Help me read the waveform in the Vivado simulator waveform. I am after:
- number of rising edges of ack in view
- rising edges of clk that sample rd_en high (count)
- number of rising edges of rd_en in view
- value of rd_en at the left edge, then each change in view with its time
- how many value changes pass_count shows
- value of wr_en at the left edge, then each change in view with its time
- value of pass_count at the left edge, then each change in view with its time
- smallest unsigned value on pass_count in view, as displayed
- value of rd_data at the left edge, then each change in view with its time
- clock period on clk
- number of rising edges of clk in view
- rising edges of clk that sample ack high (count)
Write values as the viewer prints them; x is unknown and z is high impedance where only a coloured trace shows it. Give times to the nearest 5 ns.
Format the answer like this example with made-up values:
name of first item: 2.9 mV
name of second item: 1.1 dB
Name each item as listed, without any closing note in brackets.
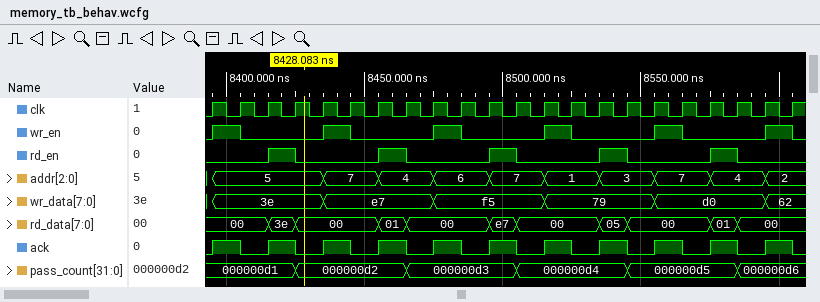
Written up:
number of rising edges of ack in view: 11
rising edges of clk that sample rd_en high: 5
number of rising edges of rd_en in view: 5
value of rd_en at the left edge, then each change in view with its time: 0, 1 at 8415 ns, 0 at 8425 ns, 1 at 8455 ns, 0 at 8465 ns, 1 at 8495 ns, 0 at 8505 ns, 1 at 8535 ns, 0 at 8545 ns, 1 at 8575 ns, 0 at 8585 ns
how many value changes pass_count shows: 5
value of wr_en at the left edge, then each change in view with its time: 0, 1 at 8395 ns, 0 at 8405 ns, 1 at 8435 ns, 0 at 8445 ns, 1 at 8475 ns, 0 at 8485 ns, 1 at 8515 ns, 0 at 8525 ns, 1 at 8555 ns, 0 at 8565 ns, 1 at 8595 ns, 0 at 8605 ns
value of pass_count at the left edge, then each change in view with its time: 000000d1, 000000d2 at 8425 ns, 000000d3 at 8465 ns, 000000d4 at 8505 ns, 000000d5 at 8545 ns, 000000d6 at 8585 ns
smallest unsigned value on pass_count in view, as displayed: 000000d1
value of rd_data at the left edge, then each change in view with its time: 00, 3e at 8415 ns, 00 at 8425 ns, 01 at 8455 ns, 00 at 8465 ns, e7 at 8495 ns, 00 at 8505 ns, 05 at 8535 ns, 00 at 8545 ns, 01 at 8575 ns, 00 at 8585 ns
clock period on clk: 10 ns
number of rising edges of clk in view: 22
rising edges of clk that sample ack high: 11
